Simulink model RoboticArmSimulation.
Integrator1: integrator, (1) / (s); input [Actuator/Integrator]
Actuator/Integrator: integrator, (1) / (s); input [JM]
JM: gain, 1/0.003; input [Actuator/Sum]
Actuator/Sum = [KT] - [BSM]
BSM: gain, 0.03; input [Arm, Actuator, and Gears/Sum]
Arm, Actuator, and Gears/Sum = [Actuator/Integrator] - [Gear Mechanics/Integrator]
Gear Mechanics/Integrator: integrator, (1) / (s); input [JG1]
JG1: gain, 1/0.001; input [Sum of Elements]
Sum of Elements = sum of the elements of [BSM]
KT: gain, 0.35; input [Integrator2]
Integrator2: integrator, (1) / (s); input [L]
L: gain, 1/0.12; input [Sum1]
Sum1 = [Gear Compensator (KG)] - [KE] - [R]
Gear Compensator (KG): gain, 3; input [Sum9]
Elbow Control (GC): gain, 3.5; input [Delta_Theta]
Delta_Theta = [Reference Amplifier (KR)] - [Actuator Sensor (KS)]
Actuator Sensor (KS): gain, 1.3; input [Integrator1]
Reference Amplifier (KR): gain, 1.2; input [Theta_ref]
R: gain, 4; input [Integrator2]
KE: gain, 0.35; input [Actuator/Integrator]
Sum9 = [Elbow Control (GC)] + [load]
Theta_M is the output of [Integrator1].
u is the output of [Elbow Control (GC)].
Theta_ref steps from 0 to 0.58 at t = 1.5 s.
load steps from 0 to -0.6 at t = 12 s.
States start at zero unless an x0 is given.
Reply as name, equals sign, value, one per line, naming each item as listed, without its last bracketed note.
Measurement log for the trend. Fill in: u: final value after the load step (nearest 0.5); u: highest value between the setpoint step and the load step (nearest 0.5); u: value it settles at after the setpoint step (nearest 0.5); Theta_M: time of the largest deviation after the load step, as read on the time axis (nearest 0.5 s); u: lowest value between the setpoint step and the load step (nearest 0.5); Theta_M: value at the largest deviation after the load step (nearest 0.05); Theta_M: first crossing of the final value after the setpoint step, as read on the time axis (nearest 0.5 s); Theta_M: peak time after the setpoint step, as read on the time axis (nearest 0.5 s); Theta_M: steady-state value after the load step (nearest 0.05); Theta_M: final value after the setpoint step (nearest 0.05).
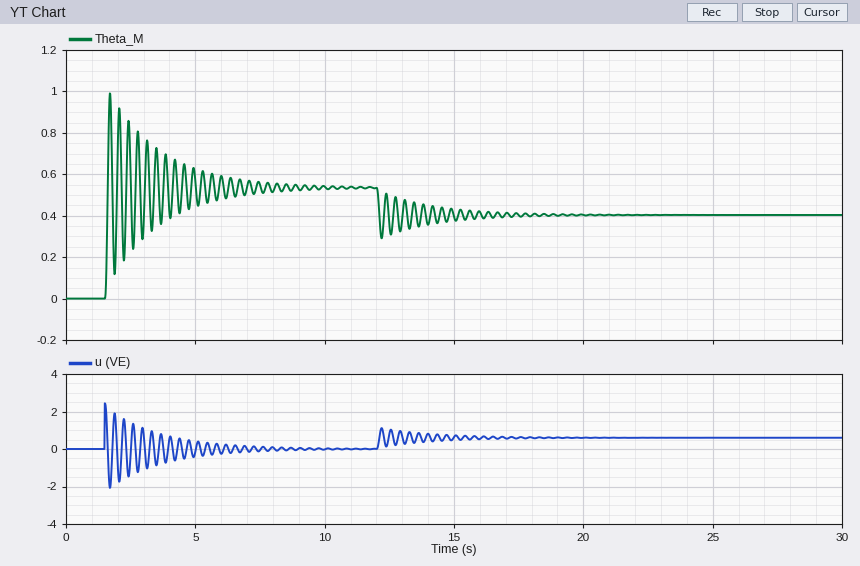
u: final value after the load step = 0.5
u: highest value between the setpoint step and the load step = 2.5
u: value it settles at after the setpoint step = 0.0
Theta_M: time of the largest deviation after the load step, as read on the time axis = 12.0 s
u: lowest value between the setpoint step and the load step = -2.0
Theta_M: value at the largest deviation after the load step = 0.30
Theta_M: first crossing of the final value after the setpoint step, as read on the time axis = 1.5 s
Theta_M: peak time after the setpoint step, as read on the time axis = 1.5 s
Theta_M: steady-state value after the load step = 0.40
Theta_M: final value after the setpoint step = 0.55
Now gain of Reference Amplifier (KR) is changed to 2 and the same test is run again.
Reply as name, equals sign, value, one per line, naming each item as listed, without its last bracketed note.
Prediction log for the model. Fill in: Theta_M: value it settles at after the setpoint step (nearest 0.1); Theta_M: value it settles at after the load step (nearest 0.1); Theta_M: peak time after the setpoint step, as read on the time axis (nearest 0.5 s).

Theta_M: value it settles at after the setpoint step = 0.9
Theta_M: value it settles at after the load step = 0.8
Theta_M: peak time after the setpoint step, as read on the time axis = 1.5 s
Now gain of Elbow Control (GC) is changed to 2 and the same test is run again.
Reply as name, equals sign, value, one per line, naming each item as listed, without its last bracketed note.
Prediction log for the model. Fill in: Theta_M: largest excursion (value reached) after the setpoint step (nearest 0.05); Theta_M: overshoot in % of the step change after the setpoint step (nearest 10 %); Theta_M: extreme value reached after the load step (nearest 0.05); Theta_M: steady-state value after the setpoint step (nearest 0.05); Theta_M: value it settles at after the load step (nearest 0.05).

Theta_M: largest excursion (value reached) after the setpoint step = 0.85
Theta_M: overshoot in % of the step change after the setpoint step = 60 %
Theta_M: extreme value reached after the load step = 0.15
Theta_M: steady-state value after the setpoint step = 0.55
Theta_M: value it settles at after the load step = 0.30
